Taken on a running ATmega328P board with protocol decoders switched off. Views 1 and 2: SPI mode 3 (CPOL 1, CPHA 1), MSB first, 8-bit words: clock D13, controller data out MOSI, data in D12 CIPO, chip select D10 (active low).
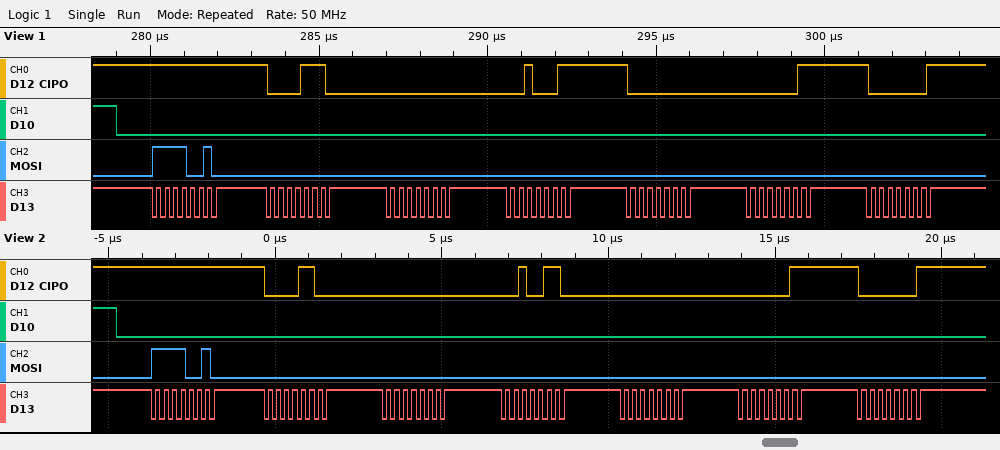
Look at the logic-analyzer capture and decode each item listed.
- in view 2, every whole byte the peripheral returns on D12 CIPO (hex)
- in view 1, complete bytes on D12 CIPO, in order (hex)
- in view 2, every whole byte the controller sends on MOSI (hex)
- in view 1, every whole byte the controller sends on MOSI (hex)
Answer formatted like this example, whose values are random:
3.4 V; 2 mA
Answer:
FF 0C 00 26 00 03 01; FF 0E 00 23 00 03 01; F2 00 00 00 00 00 00; F2 00 00 00 00 00 00
